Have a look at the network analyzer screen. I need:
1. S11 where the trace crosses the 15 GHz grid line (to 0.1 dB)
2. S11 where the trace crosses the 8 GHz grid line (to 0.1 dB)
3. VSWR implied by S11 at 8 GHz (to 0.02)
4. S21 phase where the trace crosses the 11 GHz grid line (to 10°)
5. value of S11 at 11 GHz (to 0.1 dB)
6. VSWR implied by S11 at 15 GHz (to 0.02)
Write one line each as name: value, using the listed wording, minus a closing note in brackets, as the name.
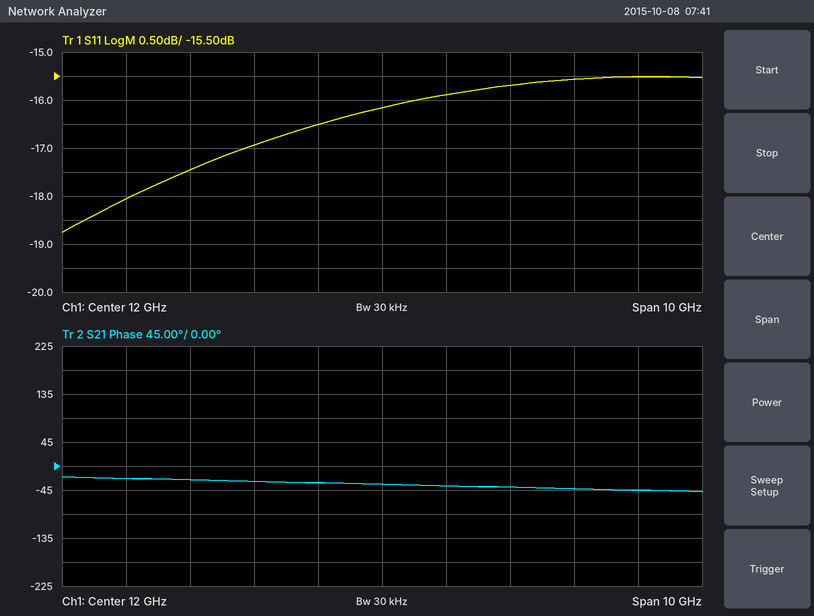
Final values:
S11 where the trace crosses the 15 GHz grid line: -15.6 dB
S11 where the trace crosses the 8 GHz grid line: -18.1 dB
VSWR implied by S11 at 8 GHz: 1.28
S21 phase where the trace crosses the 11 GHz grid line: -30°
value of S11 at 11 GHz: -16.5 dB
VSWR implied by S11 at 15 GHz: 1.40
